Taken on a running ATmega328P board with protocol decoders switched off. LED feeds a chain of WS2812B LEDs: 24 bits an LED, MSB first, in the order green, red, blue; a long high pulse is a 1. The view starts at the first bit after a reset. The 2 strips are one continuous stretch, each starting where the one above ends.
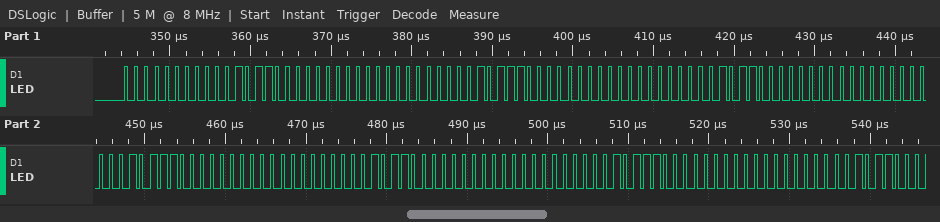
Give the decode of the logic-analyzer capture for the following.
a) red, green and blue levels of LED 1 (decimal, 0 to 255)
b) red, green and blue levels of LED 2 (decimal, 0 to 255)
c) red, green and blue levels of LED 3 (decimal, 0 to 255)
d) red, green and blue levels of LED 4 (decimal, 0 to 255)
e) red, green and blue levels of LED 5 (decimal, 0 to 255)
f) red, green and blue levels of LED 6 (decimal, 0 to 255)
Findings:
22, 0, 0
23, 0, 0
22, 0, 0
23, 0, 0
22, 0, 0
23, 0, 0
